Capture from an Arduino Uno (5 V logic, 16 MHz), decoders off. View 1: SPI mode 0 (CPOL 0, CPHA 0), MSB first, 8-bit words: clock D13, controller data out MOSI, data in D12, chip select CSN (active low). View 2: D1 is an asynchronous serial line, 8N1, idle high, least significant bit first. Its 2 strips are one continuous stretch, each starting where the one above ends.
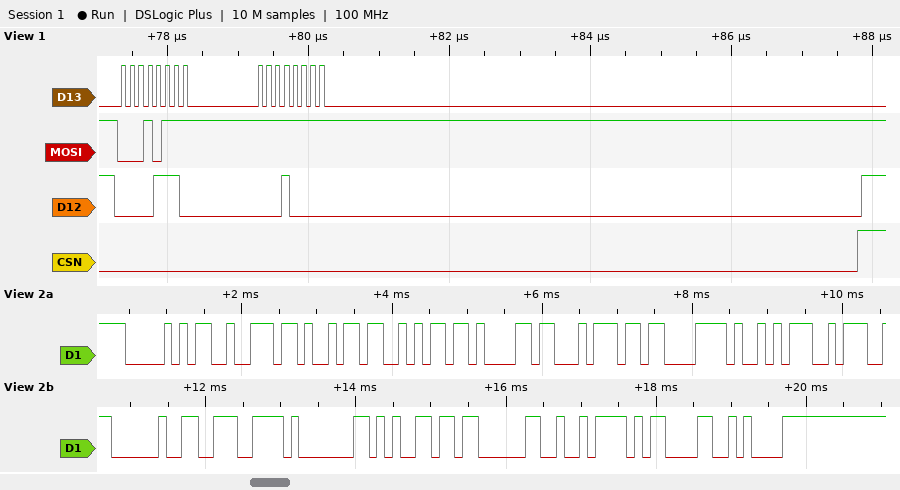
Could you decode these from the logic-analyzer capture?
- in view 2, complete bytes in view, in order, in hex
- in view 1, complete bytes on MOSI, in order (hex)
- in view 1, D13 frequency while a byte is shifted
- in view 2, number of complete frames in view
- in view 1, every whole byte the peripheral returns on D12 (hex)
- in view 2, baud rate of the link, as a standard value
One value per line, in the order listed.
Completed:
50 72 69 6A 61 74 C3 A9 3A 20 CE 01 65 03 D2 0D 0A
17 FF
8 MHz
17
0E 10
9600 baud
